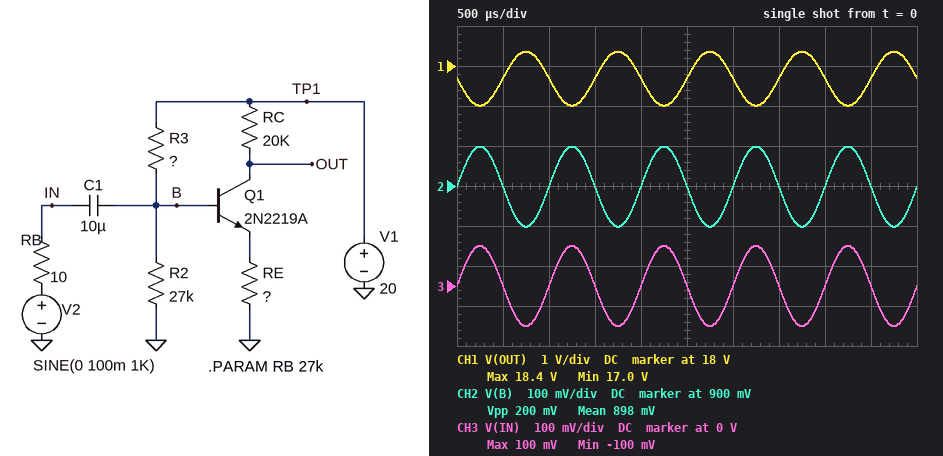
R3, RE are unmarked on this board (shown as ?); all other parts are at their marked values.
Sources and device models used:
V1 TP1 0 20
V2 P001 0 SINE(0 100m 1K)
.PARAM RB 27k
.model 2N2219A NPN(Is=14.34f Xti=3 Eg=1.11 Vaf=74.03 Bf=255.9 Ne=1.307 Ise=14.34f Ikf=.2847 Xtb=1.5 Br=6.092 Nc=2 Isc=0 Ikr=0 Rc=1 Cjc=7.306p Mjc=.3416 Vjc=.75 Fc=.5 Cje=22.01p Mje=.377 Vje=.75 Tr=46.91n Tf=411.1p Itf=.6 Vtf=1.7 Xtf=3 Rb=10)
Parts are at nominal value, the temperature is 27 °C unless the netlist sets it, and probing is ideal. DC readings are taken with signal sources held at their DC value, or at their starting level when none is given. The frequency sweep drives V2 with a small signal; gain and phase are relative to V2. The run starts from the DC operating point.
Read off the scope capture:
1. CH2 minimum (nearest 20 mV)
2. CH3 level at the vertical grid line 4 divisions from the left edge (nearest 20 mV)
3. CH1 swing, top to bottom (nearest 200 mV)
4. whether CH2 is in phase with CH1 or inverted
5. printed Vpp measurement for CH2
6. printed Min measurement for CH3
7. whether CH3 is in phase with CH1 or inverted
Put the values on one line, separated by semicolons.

800 mV; 0 V; 1.4 V; inverted; 200 mV; -100 mV; inverted
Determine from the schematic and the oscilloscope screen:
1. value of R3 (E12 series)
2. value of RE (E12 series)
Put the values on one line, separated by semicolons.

560 kΩ; 2.7 kΩ
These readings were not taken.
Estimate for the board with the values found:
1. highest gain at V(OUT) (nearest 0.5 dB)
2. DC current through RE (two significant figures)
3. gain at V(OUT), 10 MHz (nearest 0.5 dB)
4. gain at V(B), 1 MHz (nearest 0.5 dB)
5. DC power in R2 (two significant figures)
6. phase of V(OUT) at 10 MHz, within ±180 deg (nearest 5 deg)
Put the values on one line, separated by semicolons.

16.5 dB; 120 µA; 7.5 dB; 0 dB; 30 µW; 60 deg
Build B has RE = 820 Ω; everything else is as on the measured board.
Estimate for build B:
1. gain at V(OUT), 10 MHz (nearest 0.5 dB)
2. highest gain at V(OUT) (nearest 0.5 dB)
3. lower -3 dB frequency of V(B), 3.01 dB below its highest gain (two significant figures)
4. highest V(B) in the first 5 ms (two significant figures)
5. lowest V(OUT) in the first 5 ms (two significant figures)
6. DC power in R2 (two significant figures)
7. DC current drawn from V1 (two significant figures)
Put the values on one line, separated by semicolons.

16.0 dB; 27.0 dB; 730 mHz; 970 mV; 12 V; 28 µW; 340 µA
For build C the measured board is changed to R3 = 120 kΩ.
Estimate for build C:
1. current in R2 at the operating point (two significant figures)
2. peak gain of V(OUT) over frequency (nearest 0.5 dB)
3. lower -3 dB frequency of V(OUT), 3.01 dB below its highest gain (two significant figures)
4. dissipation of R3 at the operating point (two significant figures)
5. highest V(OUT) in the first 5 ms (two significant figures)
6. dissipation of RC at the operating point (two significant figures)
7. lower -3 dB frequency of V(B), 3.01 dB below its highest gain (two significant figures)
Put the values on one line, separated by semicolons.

110 µA; 0 dB; 390 kHz; 2.4 mW; 2.8 V; 15 mW; 6.6 Hz
